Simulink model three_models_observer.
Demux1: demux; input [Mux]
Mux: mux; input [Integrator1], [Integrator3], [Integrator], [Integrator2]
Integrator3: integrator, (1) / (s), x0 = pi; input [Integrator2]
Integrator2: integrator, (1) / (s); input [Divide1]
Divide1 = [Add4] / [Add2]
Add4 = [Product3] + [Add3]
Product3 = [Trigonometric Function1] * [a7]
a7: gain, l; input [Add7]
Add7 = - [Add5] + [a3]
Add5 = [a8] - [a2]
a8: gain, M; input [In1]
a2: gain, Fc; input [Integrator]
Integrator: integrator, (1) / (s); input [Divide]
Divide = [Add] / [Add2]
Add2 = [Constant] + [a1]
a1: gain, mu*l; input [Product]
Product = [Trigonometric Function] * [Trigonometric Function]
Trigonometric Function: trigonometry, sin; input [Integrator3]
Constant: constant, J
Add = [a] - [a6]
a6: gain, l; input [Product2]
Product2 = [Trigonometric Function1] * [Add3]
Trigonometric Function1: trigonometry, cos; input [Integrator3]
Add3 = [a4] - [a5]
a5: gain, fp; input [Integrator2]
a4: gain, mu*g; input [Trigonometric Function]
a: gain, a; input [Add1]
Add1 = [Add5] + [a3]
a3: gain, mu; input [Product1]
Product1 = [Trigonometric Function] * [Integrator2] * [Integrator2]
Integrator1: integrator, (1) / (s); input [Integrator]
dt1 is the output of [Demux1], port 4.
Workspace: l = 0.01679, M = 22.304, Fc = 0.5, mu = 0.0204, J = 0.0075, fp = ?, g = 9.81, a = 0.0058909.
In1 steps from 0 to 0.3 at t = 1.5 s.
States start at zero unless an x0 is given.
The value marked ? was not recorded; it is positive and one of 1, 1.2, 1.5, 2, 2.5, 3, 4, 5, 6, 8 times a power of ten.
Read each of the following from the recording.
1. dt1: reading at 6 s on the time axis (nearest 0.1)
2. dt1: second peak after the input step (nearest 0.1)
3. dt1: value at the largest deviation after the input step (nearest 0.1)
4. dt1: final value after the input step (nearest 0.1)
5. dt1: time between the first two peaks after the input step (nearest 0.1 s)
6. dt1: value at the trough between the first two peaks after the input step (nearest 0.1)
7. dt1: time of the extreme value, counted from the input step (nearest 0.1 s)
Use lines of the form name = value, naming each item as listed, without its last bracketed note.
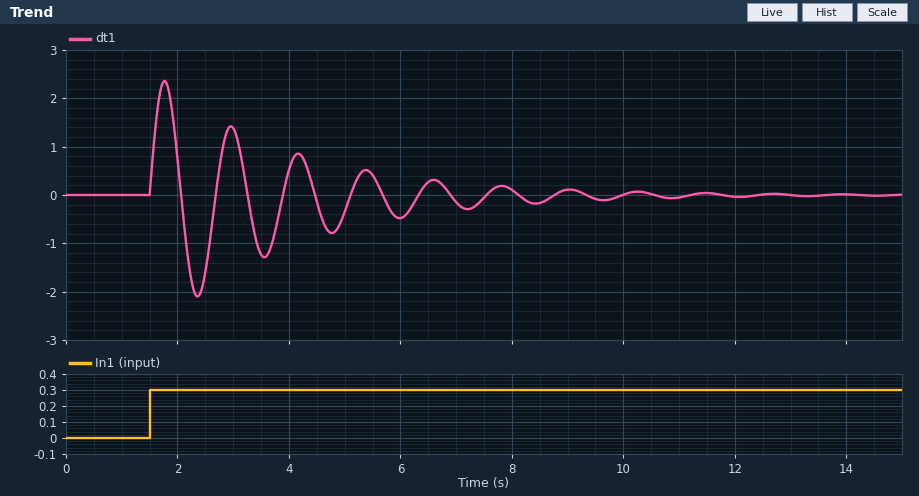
dt1: reading at 6 s on the time axis = -0.5
dt1: second peak after the input step = 1.4
dt1: value at the largest deviation after the input step = 2.4
dt1: final value after the input step = 0.0
dt1: time between the first two peaks after the input step = 1.2 s
dt1: value at the trough between the first two peaks after the input step = -2.1
dt1: time of the extreme value, counted from the input step = 0.3 s
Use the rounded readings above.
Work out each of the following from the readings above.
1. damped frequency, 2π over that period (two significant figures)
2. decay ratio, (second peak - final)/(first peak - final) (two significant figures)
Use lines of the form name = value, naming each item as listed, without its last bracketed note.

damped frequency, 2π over that period = 5.2 rad/s
decay ratio, (second peak - final)/(first peak - final) = 0.58
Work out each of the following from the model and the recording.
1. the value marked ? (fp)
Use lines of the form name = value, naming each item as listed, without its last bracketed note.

the value marked ? = 0.006
